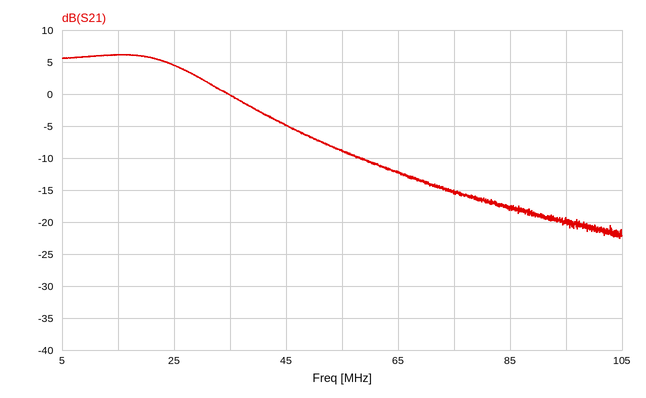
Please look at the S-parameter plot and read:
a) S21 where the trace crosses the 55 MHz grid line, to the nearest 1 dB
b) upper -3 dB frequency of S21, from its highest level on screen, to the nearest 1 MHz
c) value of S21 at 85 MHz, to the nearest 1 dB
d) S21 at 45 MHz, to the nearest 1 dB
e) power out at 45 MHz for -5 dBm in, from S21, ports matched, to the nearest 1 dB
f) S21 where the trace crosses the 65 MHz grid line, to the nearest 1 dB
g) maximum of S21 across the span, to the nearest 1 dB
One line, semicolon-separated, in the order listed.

-9 dB; 28 MHz; -18 dB; -5 dB; -10 dBm; -12 dB; 6 dB
